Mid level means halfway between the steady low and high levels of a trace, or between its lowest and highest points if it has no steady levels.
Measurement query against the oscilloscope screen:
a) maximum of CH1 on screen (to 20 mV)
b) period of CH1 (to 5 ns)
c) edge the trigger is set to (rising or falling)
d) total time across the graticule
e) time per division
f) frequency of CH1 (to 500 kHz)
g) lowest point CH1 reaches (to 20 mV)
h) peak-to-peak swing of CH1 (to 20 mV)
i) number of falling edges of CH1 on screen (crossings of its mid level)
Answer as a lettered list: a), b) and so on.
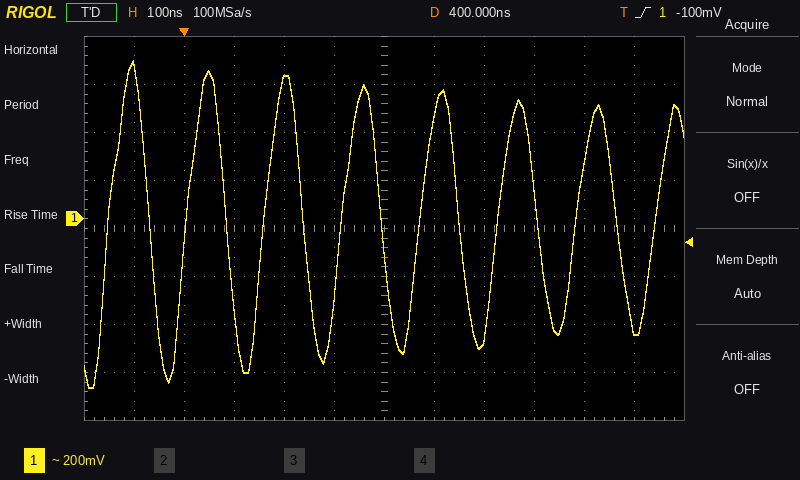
a) 660 mV
b) 155 ns
c) rising
d) 1.2 µs
e) 100 ns
f) 6.5 MHz
g) -700 mV
h) 1.36 V
i) 7
